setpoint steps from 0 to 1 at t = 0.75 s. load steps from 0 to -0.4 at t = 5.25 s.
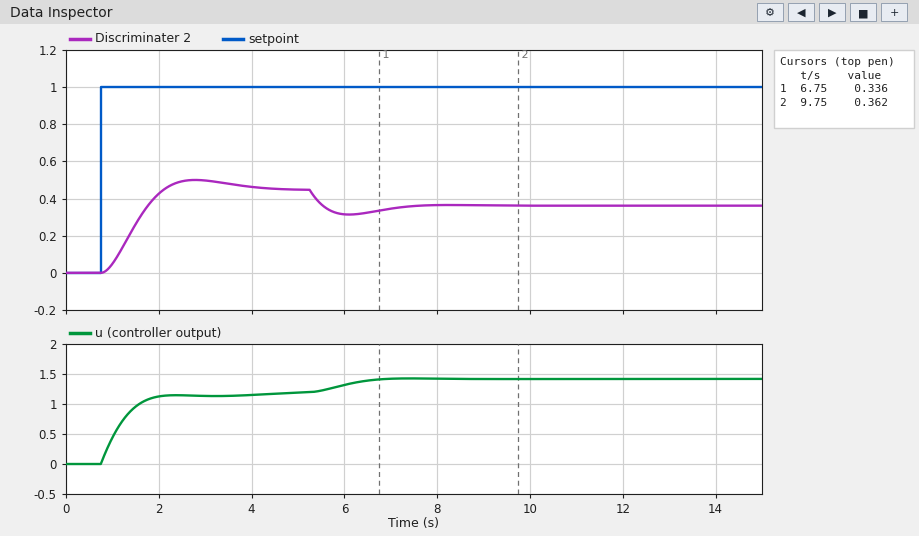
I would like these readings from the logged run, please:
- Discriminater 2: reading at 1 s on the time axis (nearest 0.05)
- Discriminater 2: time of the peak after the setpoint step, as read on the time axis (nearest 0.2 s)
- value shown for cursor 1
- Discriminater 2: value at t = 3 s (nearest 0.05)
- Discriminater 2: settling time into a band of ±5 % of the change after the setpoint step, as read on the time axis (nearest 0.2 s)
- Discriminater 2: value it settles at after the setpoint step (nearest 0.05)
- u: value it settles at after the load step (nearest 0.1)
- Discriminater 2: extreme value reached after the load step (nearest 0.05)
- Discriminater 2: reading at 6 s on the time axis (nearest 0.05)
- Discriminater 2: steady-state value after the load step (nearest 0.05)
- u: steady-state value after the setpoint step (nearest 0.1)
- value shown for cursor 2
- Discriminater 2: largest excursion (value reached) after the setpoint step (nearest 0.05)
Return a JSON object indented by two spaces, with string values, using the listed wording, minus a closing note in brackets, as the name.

{
  "Discriminater 2: reading at 1 s on the time axis": "0.05",
  "Discriminater 2: time of the peak after the setpoint step, as read on the time axis": "2.8 s",
  "value shown for cursor 1": "0.336",
  "Discriminater 2: value at t = 3 s": "0.50",
  "Discriminater 2: settling time into a band of ±5 % of the change after the setpoint step, as read on the time axis": "3.8 s",
  "Discriminater 2: value it settles at after the setpoint step": "0.45",
  "u: value it settles at after the load step": "1.4",
  "Discriminater 2: extreme value reached after the load step": "0.30",
  "Discriminater 2: reading at 6 s on the time axis": "0.30",
  "Discriminater 2: steady-state value after the load step": "0.35",
  "u: steady-state value after the setpoint step": "1.2",
  "value shown for cursor 2": "0.362",
  "Discriminater 2: largest excursion (value reached) after the setpoint step": "0.50"
}
